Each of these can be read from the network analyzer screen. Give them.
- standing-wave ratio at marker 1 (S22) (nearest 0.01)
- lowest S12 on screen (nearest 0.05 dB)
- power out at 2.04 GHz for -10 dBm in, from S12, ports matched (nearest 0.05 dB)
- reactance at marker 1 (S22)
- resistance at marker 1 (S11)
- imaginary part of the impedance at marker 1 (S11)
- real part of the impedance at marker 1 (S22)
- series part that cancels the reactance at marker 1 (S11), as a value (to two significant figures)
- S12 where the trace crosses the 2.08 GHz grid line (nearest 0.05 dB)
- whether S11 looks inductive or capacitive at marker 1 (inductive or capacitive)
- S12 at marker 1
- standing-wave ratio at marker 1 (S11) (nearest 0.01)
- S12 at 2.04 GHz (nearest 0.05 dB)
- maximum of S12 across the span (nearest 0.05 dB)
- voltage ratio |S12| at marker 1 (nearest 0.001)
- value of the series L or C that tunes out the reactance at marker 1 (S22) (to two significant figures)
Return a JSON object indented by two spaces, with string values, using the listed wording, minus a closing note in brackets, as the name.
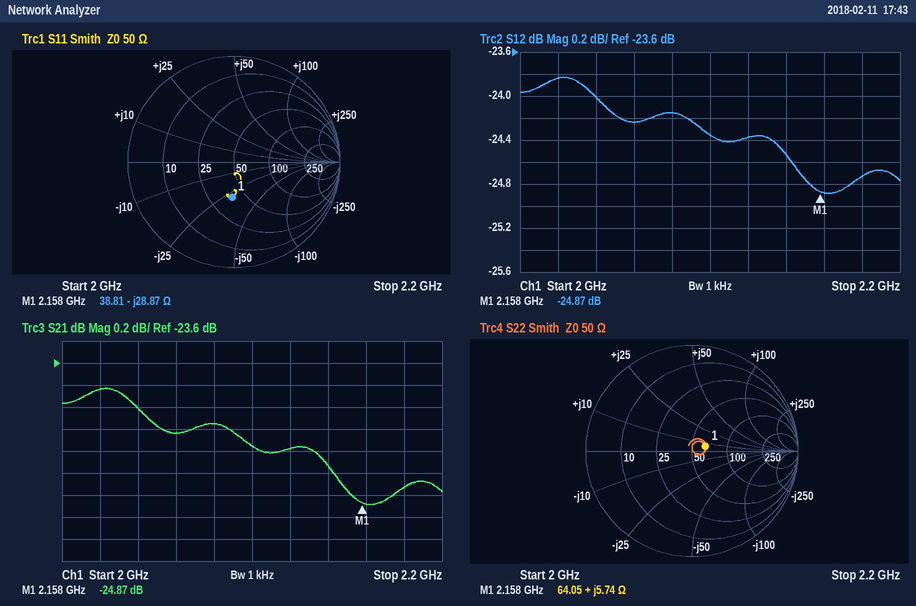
{
  "standing-wave ratio at marker 1 (S22)": "1.31",
  "lowest S12 on screen": "-24.90 dB",
  "power out at 2.04 GHz for -10 dBm in, from S12, ports matched": "-34.00 dBm",
  "reactance at marker 1": "+5.74 Ω",
  "resistance at marker 1": "38.81 Ω",
  "imaginary part of the impedance at marker 1": "-28.87 Ω",
  "real part of the impedance at marker 1": "64.05 Ω",
  "series part that cancels the reactance at marker 1 (S11), as a value": "2.1 nH",
  "S12 where the trace crosses the 2.08 GHz grid line": "-24.15 dB",
  "whether S11 looks inductive or capacitive at marker 1": "capacitive",
  "S12 at marker 1": "-24.87 dB",
  "standing-wave ratio at marker 1 (S11)": "1.99",
  "S12 at 2.04 GHz": "-24.00 dB",
  "maximum of S12 across the span": "-23.85 dB",
  "voltage ratio |S12| at marker 1": "0.057",
  "value of the series L or C that tunes out the reactance at marker 1 (S22)": "13 pF"
}
